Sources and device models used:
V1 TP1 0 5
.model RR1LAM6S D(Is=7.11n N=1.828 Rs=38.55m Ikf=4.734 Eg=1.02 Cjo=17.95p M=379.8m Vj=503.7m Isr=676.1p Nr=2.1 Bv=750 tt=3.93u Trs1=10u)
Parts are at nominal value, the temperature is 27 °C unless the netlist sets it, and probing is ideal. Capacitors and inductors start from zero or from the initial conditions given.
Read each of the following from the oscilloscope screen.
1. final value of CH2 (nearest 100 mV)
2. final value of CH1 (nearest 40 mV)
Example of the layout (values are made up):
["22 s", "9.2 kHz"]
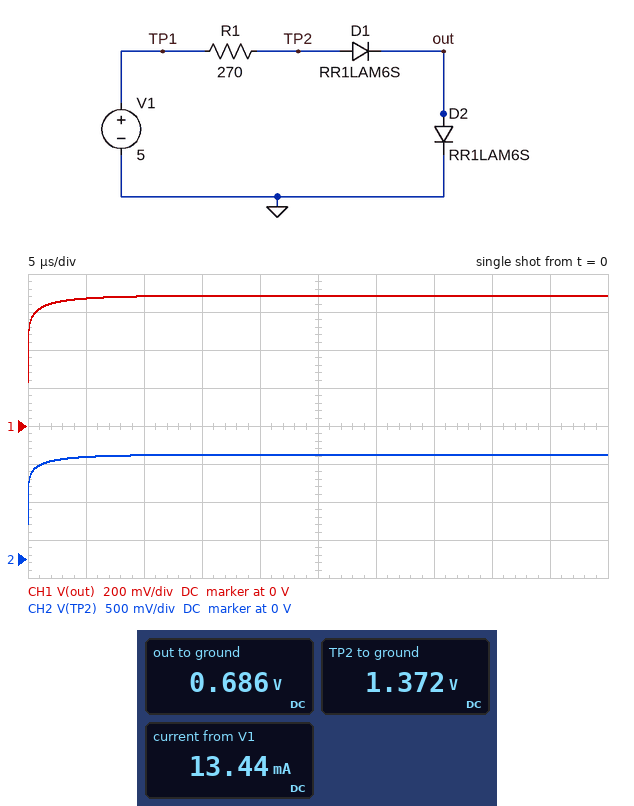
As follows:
["1.4 V", "680 mV"]
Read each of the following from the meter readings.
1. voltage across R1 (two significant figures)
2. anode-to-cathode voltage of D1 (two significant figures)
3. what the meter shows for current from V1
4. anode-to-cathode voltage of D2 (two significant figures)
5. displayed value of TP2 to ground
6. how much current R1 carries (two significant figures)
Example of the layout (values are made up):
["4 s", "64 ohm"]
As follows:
["3.6 V", "690 mV", "13.44 mA", "690 mV", "1.372 V", "13 mA"]
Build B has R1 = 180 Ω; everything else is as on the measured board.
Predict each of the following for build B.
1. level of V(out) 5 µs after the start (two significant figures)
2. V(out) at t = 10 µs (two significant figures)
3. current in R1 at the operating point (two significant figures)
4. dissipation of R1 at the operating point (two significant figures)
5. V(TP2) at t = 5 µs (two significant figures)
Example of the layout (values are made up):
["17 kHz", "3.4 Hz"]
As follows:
["690 mV", "700 mV", "20 mA", "72 mW", "1.4 V"]
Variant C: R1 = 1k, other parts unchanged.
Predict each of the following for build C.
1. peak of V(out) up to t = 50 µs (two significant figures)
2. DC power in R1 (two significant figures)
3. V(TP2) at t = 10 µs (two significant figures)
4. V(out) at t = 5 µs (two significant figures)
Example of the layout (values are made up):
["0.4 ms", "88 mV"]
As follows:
["620 mV", "14 mW", "1.2 V", "610 mV"]
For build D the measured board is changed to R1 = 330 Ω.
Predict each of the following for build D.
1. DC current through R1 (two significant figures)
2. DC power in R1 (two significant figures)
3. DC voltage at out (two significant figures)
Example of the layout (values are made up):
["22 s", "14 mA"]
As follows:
["11 mA", "40 mW", "680 mV"]
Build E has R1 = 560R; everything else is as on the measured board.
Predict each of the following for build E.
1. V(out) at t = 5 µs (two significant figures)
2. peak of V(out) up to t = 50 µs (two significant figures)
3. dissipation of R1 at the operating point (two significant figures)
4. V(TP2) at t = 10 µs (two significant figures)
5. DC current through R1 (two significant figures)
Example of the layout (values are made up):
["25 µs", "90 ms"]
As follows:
["640 mV", "650 mV", "24 mW", "1.3 V", "6.6 mA"]
